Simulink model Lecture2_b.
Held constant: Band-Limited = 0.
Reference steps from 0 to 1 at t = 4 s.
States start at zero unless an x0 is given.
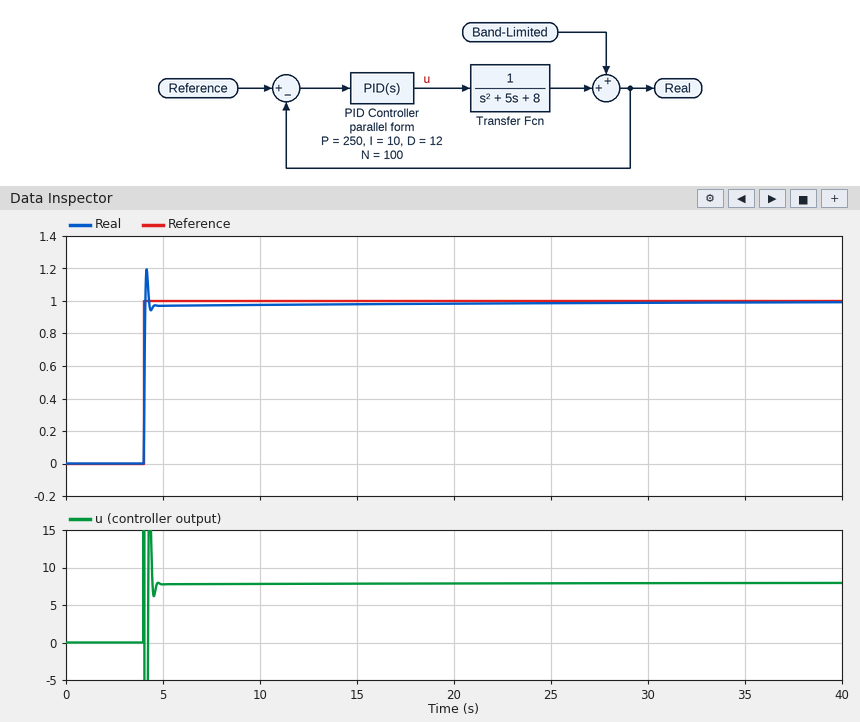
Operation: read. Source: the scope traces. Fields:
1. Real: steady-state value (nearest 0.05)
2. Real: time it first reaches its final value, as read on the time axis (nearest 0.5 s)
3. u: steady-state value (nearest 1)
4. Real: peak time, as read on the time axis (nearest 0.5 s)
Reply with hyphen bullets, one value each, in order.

- 1.00
- 4.0 s
- 8
- 4.0 s
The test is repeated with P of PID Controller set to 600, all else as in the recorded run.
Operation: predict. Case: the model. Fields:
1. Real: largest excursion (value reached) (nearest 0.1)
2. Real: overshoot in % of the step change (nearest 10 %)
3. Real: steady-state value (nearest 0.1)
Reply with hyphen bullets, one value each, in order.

- 1.4
- 40 %
- 1.0
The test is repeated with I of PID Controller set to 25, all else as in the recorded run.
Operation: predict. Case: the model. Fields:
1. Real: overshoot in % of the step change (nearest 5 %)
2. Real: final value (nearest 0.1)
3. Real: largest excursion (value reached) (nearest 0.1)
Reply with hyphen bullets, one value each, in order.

- 20 %
- 1.0
- 1.2
